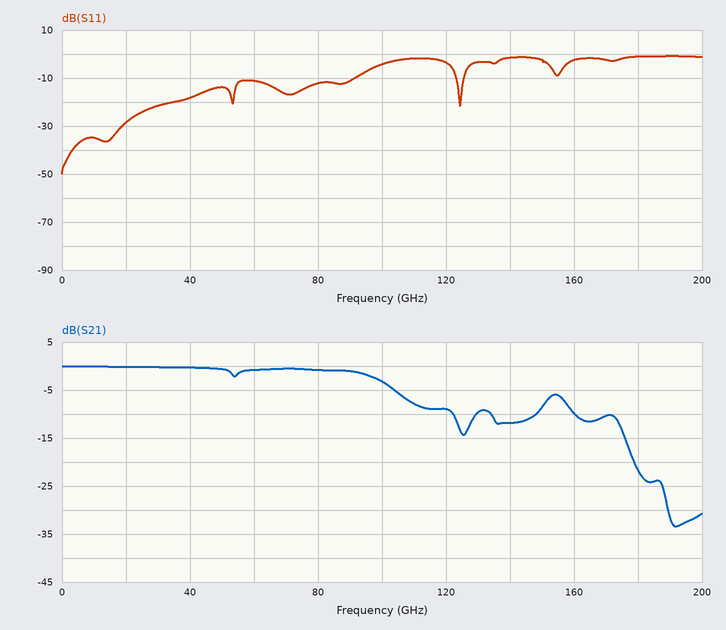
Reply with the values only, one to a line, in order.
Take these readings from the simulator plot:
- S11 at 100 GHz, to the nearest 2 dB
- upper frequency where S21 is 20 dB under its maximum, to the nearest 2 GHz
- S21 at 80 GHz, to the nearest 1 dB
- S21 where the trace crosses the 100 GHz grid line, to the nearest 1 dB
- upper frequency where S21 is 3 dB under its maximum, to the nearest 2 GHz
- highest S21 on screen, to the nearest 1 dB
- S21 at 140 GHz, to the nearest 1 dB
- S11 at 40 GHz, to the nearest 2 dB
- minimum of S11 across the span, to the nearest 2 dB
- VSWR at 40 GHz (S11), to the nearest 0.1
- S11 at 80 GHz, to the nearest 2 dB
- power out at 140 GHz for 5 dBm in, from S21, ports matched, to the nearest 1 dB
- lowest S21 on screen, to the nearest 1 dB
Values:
-4 dB
178 GHz
-1 dB
-3 dB
100 GHz
0 dB
-12 dB
-18 dB
-50 dB
1.3
-12 dB
-7 dBm
-33 dB
